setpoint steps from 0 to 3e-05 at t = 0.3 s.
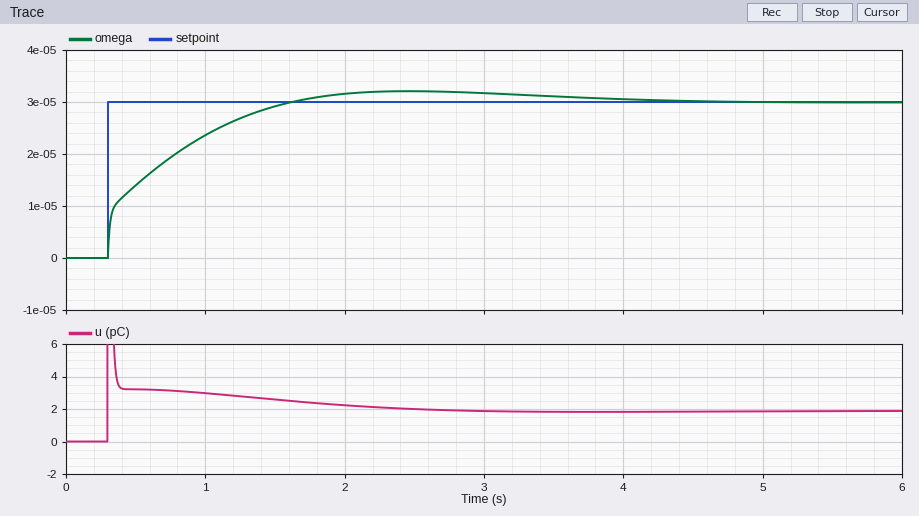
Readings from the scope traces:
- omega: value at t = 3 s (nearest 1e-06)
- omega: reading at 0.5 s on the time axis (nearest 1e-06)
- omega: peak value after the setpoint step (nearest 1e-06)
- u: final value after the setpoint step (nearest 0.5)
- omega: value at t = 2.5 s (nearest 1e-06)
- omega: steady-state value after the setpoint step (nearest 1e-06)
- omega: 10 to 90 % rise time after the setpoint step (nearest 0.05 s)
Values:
0.000032
0.000014
0.000032
2.0
0.000032
0.000030
0.95 s
